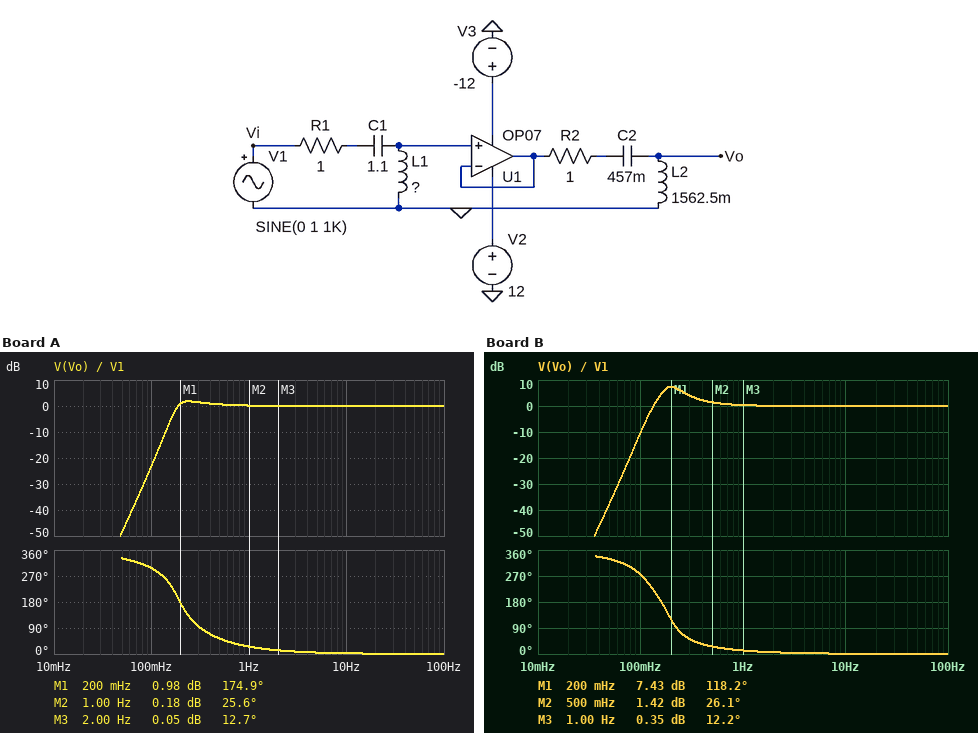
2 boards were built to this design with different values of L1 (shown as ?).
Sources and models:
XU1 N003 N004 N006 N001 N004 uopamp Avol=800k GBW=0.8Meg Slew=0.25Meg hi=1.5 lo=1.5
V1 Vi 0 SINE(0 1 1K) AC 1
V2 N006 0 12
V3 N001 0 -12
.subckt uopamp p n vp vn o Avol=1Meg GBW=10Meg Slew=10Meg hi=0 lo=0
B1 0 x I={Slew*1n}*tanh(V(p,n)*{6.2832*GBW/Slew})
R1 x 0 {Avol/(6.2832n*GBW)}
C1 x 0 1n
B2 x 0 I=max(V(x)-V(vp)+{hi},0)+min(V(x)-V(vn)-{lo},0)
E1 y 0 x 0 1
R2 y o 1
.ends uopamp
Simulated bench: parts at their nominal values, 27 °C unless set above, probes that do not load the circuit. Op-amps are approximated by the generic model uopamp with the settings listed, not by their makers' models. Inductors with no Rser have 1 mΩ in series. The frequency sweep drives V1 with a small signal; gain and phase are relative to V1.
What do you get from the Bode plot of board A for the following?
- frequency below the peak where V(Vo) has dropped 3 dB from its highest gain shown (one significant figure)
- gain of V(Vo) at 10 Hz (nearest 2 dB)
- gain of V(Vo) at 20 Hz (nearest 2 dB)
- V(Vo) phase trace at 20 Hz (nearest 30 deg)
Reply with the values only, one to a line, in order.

200 mHz
0 dB
0 dB
0 deg
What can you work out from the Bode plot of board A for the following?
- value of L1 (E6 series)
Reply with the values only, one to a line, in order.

470 mH
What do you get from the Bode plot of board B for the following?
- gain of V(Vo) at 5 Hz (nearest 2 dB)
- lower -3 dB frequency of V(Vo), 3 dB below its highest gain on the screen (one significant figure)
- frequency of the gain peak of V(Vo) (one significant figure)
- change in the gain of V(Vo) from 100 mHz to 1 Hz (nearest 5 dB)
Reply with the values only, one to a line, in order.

0 dB
200 mHz
200 mHz
10 dB
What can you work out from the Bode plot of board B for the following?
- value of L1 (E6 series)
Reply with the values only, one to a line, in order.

1.5 H
